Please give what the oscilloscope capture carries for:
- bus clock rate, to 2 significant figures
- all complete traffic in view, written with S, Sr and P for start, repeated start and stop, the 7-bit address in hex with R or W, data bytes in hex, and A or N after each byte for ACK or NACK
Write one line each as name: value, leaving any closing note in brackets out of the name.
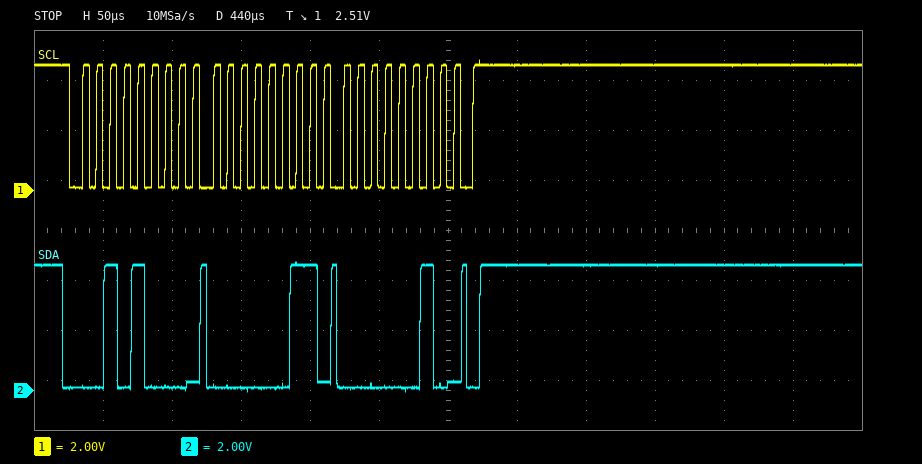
bus clock rate, to 2 significant figures: 100 kHz
all complete traffic in view, written with S, Sr and P for start, repeated start and stop, the 7-bit address in hex with R or W, data bytes in hex, and A or N after each byte for ACK or NACK: S 14W A 03 A 02 A P
